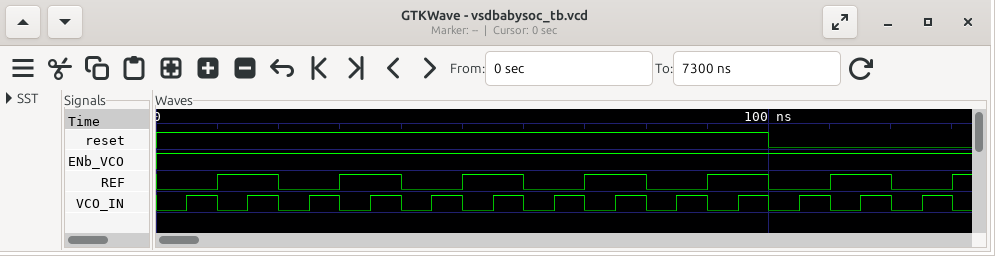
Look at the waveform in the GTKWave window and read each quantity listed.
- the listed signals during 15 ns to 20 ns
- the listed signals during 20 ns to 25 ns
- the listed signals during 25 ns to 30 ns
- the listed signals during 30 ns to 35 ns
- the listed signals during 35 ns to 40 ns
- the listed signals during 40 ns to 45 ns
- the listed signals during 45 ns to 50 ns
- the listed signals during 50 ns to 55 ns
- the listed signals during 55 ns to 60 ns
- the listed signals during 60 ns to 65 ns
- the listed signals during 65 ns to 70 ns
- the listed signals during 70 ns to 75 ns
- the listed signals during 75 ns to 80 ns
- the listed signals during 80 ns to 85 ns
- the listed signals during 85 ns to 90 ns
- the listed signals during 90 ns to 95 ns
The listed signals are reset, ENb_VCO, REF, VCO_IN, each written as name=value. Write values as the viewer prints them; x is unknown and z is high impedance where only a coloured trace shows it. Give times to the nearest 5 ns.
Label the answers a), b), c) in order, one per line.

a) reset=1, ENb_VCO=1, REF=1, VCO_IN=1
b) reset=1, ENb_VCO=1, REF=0, VCO_IN=0
c) reset=1, ENb_VCO=1, REF=0, VCO_IN=1
d) reset=1, ENb_VCO=1, REF=1, VCO_IN=0
e) reset=1, ENb_VCO=1, REF=1, VCO_IN=1
f) reset=1, ENb_VCO=1, REF=0, VCO_IN=0
g) reset=1, ENb_VCO=1, REF=0, VCO_IN=1
h) reset=1, ENb_VCO=1, REF=1, VCO_IN=0
i) reset=1, ENb_VCO=1, REF=1, VCO_IN=1
j) reset=1, ENb_VCO=1, REF=0, VCO_IN=0
k) reset=1, ENb_VCO=1, REF=0, VCO_IN=1
l) reset=1, ENb_VCO=1, REF=1, VCO_IN=0
m) reset=1, ENb_VCO=1, REF=1, VCO_IN=1
n) reset=1, ENb_VCO=1, REF=0, VCO_IN=0
o) reset=1, ENb_VCO=1, REF=0, VCO_IN=1
p) reset=1, ENb_VCO=1, REF=1, VCO_IN=0
